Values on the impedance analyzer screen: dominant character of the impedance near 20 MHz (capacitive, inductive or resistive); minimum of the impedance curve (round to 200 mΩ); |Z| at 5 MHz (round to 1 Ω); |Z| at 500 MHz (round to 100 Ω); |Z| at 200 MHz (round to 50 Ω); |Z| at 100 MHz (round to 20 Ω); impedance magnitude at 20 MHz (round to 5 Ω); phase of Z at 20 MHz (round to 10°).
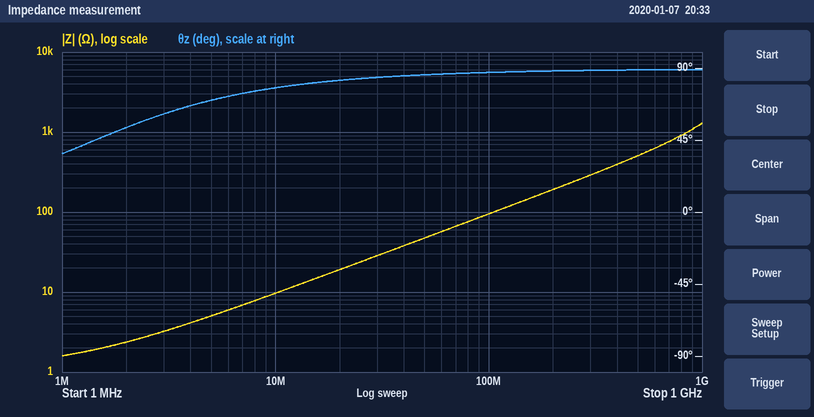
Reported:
inductive
1.6 Ω
5 Ω
500 Ω
200 Ω
100 Ω
20 Ω
80°
